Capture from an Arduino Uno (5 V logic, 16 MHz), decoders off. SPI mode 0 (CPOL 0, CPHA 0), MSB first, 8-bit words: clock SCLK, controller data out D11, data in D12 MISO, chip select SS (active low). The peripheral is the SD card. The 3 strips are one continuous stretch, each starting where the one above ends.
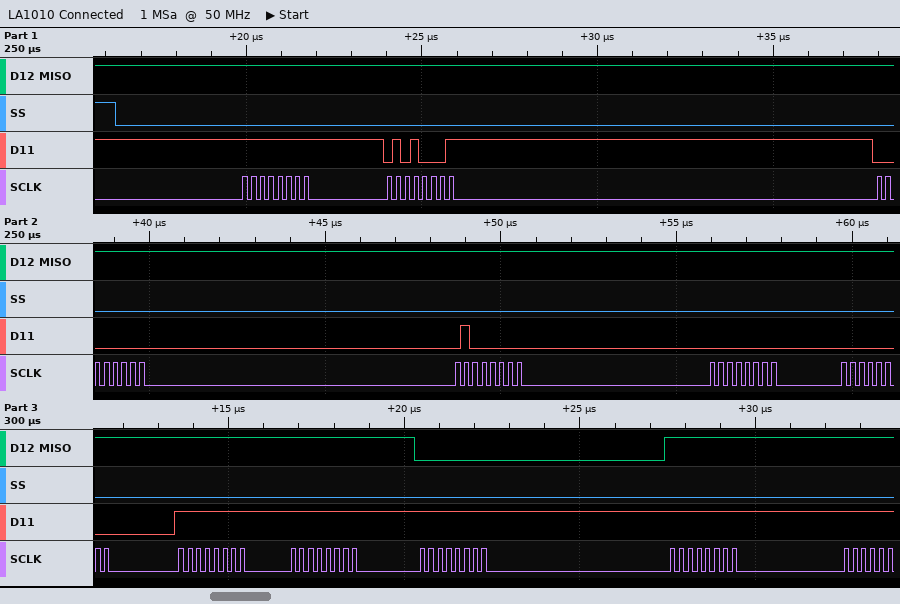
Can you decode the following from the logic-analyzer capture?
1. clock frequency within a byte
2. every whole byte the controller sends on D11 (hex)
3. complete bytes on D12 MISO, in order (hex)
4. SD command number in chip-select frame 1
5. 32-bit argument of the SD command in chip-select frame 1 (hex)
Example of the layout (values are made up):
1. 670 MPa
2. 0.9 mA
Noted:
1. 4 MHz
2. 0xFF 0x51 0x00 0x40 0x00 0x00 0xFF 0xFF 0xFF 0xFF
3. 0xFF 0xFF 0xFF 0xFF 0xFF 0xFF 0xFF 0xFF 0x00 0xFF
4. CMD17
5. 0x00400000
